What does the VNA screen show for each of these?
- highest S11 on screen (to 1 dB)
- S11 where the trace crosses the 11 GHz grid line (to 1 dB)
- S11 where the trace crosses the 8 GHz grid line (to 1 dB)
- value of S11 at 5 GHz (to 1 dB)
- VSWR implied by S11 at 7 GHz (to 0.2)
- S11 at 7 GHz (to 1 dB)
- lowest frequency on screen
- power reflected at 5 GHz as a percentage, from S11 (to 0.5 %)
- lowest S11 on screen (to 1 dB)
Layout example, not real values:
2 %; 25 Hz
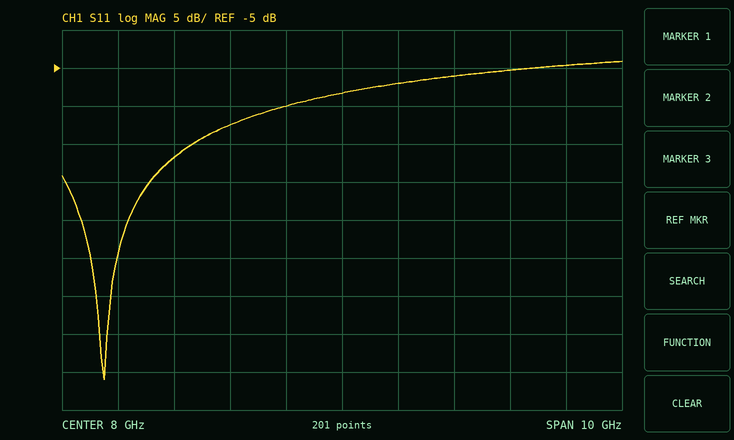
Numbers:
-4 dB; -5 dB; -8 dB; -17 dB; 2.0; -10 dB; 3 GHz; 2.0 %; -46 dB
